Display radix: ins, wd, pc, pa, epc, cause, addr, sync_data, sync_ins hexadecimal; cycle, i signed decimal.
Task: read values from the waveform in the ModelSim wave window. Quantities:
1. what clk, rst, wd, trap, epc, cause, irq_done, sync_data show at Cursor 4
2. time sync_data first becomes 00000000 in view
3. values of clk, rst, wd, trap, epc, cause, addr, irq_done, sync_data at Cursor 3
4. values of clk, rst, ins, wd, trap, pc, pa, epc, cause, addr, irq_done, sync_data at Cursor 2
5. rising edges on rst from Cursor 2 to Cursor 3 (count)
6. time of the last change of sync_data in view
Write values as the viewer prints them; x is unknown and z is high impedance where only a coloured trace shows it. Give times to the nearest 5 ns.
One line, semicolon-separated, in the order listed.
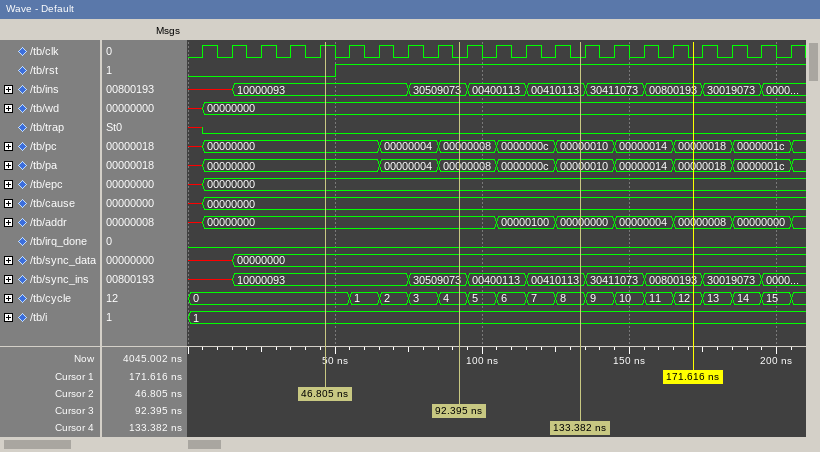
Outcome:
clk=0, rst=1, wd=00000000, trap=0, epc=00000000, cause=00000000, irq_done=0, sync_data=00000000; 15 ns; clk=0, rst=1, wd=00000000, trap=0, epc=00000000, cause=00000000, addr=00000000, irq_done=0, sync_data=00000000; clk=1, rst=0, ins=10000093, wd=00000000, trap=0, pc=00000000, pa=00000000, epc=00000000, cause=00000000, addr=00000000, irq_done=0, sync_data=00000000; 1; 15 ns
